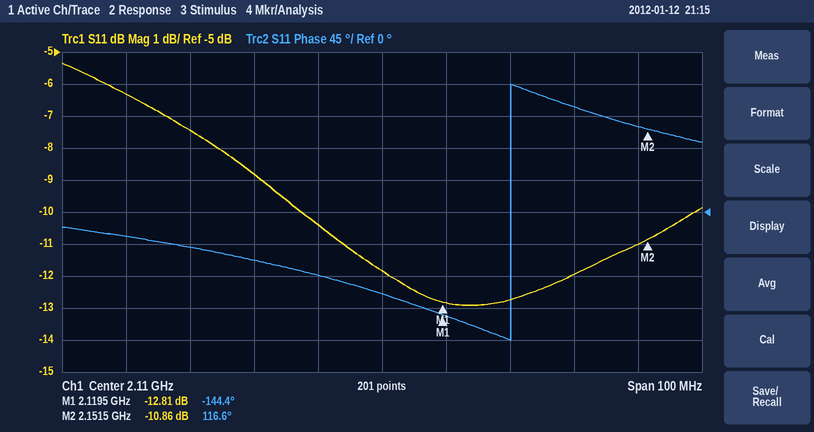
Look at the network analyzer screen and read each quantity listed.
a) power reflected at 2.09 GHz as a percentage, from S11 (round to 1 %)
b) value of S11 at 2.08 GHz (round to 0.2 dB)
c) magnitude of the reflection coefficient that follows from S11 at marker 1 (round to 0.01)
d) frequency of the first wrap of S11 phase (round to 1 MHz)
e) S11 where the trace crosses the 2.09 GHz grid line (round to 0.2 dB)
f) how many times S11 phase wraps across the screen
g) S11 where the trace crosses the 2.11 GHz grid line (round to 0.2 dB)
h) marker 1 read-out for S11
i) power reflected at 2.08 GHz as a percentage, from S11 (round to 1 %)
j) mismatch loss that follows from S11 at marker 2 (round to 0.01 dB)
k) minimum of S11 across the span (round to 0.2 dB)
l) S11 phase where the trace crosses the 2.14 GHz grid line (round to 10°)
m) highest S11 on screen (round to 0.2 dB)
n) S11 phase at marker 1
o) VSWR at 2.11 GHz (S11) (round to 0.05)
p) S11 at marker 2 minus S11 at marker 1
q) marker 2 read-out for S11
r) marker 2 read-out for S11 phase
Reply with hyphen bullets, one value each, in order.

- 13 %
- -7.4 dB
- 0.23
- 2.130 GHz
- -8.8 dB
- 1
- -11.8 dB
- -12.81 dB
- 18 %
- 0.37 dB
- -13.0 dB
- 150°
- -5.4 dB
- -144.4°
- 1.70
- 1.95 dB
- -10.86 dB
- 116.6°
